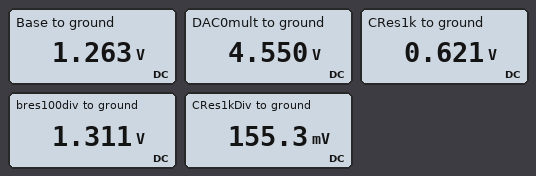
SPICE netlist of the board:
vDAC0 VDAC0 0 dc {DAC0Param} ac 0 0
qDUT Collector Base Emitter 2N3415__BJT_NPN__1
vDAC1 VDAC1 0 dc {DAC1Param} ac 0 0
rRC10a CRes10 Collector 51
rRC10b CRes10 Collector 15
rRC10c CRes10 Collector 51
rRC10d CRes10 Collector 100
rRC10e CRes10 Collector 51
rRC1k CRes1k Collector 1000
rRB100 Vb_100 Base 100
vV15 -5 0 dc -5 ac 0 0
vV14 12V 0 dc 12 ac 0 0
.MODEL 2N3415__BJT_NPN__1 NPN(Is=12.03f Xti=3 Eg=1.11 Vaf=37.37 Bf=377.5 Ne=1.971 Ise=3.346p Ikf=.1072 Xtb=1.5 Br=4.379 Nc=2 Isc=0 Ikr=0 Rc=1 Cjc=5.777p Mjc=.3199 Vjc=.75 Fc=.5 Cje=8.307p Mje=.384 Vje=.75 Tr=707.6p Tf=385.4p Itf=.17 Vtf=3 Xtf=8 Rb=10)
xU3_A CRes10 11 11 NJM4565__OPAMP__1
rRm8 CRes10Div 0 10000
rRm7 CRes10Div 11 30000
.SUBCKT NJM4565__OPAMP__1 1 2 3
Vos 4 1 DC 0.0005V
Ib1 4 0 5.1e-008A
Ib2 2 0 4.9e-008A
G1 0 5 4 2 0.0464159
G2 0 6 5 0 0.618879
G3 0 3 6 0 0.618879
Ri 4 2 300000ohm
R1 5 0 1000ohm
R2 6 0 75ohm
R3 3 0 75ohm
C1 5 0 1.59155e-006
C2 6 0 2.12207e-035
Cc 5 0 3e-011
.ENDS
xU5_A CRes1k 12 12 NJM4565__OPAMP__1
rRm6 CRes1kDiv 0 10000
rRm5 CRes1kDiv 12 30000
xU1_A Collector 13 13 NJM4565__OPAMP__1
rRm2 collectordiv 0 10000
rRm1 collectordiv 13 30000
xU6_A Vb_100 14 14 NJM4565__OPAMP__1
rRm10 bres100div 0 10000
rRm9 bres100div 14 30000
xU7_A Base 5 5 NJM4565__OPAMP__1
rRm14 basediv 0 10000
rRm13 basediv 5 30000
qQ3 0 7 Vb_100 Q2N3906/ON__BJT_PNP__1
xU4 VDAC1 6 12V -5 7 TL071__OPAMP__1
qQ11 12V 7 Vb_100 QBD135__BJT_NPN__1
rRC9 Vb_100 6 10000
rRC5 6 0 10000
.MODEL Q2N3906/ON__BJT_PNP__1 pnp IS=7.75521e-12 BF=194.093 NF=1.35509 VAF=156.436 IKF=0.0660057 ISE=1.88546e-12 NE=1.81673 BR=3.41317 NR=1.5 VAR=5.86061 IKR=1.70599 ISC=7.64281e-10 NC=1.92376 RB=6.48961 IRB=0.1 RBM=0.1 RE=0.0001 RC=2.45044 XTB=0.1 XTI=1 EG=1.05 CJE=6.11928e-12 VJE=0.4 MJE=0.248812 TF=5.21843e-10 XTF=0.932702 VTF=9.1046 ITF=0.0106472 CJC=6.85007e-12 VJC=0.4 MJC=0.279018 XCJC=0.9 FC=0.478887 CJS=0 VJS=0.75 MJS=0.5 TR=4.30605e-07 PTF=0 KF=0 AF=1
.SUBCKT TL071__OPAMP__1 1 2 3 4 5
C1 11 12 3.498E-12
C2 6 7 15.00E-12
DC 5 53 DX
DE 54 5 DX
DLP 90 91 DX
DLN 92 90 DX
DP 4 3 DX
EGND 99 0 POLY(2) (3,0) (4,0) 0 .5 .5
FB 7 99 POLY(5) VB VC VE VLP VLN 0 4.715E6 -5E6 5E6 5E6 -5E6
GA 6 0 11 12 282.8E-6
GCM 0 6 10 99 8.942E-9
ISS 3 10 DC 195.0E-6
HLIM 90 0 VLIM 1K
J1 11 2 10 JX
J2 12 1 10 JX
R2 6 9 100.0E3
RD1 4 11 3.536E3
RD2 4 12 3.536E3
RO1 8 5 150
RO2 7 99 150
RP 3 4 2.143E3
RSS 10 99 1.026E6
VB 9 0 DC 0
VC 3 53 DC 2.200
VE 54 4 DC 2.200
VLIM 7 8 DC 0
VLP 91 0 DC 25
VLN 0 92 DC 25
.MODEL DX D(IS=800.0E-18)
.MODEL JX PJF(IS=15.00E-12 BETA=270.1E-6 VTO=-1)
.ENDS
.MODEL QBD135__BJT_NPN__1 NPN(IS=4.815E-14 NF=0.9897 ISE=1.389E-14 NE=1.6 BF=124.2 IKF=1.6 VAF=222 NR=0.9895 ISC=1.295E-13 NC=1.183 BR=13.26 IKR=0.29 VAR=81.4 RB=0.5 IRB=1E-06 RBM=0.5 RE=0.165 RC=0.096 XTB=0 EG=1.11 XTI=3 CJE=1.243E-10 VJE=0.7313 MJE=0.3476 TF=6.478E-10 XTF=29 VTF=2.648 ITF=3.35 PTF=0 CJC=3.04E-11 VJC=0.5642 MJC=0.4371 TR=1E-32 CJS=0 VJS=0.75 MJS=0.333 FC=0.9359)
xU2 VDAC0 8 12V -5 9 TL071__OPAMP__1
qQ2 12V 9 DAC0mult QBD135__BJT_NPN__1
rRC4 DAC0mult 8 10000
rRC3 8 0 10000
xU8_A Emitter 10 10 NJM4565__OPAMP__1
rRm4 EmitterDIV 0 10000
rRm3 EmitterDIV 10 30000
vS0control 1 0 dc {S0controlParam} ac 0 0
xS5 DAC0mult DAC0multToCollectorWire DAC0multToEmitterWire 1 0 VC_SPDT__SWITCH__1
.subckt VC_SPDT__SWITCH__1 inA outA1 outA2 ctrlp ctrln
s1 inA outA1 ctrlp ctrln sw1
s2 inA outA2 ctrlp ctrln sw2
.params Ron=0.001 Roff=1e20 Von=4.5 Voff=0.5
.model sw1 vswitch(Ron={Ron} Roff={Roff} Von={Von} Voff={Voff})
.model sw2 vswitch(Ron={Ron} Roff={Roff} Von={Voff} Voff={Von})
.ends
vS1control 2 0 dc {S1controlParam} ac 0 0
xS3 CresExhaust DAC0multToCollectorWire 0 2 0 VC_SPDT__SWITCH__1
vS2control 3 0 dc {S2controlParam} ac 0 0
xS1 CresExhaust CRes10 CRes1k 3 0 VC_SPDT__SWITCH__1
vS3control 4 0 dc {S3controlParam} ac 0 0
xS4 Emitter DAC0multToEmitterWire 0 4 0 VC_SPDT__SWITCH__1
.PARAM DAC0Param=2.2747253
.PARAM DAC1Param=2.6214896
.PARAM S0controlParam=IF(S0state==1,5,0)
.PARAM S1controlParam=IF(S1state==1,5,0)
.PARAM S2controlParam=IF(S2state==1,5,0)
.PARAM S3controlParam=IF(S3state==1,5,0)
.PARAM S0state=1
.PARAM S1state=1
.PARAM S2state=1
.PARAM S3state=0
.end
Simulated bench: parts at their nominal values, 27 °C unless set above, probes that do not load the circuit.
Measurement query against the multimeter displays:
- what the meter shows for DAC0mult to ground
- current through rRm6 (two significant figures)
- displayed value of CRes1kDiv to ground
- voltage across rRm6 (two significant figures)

4.550 V
16 µA
155.3 mV
160 mV
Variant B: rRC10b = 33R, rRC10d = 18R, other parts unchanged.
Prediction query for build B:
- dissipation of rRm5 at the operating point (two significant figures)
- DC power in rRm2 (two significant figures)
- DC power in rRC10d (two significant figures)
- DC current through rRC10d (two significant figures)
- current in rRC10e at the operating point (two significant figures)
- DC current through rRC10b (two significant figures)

8.1 µW
2.7 µW
840 mW
220 mA
76 mA
120 mA
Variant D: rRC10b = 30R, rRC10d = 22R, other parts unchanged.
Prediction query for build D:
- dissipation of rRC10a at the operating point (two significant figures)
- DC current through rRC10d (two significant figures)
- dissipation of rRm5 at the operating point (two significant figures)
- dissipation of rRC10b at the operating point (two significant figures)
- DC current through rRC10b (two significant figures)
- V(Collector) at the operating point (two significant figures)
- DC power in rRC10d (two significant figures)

300 mW
180 mA
7.4 µW
510 mW
130 mA
630 mV
700 mW
